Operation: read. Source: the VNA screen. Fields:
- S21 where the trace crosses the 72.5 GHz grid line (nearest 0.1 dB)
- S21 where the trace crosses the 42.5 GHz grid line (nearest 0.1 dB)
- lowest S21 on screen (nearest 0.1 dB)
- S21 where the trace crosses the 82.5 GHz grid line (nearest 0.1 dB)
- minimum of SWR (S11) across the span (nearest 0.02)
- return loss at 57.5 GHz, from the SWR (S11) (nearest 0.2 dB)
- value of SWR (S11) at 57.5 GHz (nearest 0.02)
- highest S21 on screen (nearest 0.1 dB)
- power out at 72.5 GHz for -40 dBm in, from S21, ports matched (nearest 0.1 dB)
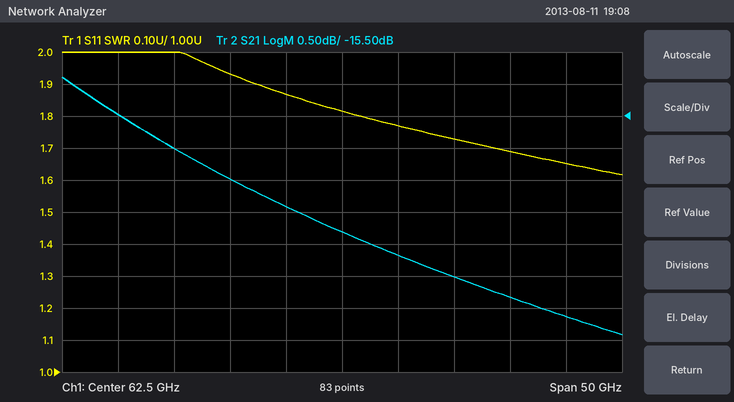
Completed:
-18.0 dB
-15.5 dB
-18.9 dB
-18.6 dB
1.62
10.4 dB
1.86
-14.9 dB
-58.0 dBm
